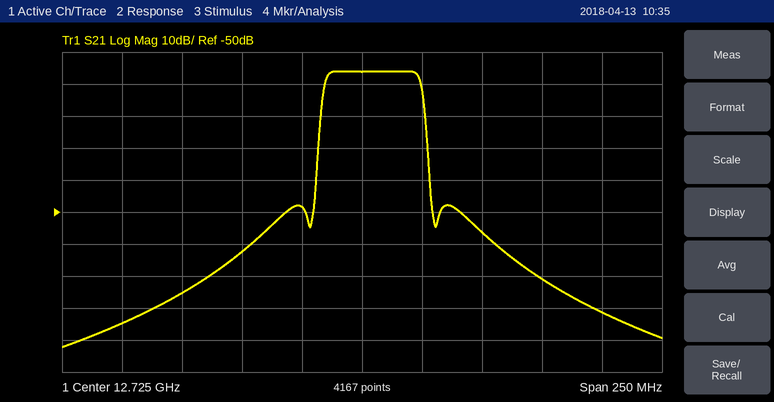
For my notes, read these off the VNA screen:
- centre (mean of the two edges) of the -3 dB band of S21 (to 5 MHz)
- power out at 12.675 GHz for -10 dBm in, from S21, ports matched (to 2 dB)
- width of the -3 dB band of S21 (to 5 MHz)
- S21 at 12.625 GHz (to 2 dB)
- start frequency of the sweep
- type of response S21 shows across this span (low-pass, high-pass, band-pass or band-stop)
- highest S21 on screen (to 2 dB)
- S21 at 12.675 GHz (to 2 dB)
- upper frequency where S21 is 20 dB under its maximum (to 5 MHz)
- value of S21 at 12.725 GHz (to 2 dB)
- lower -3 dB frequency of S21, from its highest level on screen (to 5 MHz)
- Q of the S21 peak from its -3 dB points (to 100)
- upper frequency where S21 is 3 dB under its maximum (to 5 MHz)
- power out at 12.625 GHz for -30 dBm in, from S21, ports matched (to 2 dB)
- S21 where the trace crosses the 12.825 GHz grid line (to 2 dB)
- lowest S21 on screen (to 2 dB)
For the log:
12.730 GHz
-72 dBm
40 MHz
-84 dB
12.6 GHz
band-pass
-6 dB
-62 dB
12.750 GHz
-6 dB
12.710 GHz
300
12.750 GHz
-114 dBm
-82 dB
-92 dB
